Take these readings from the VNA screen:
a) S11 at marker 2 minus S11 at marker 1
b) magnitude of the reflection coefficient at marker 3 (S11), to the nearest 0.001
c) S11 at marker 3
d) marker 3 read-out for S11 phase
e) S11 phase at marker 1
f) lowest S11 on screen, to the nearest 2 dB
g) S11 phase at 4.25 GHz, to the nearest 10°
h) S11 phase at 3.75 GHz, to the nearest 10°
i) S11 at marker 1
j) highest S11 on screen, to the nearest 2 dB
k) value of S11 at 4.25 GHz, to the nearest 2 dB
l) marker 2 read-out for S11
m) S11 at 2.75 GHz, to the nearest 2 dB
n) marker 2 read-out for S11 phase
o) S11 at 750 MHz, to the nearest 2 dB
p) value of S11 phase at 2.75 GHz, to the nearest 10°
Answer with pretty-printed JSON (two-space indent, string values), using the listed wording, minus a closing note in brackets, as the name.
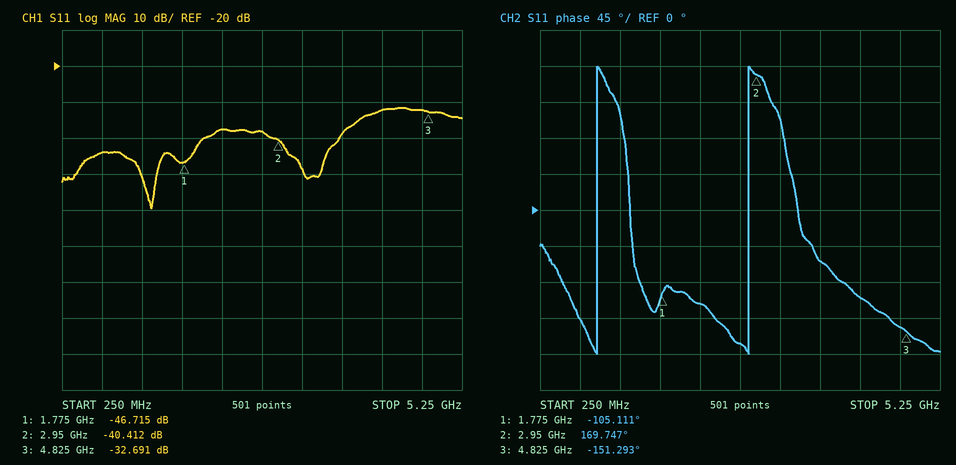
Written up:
{
  "S11 at marker 2 minus S11 at marker 1": "6.303 dB",
  "magnitude of the reflection coefficient at marker 3 (S11), to the nearest 0.001": "0.023",
  "S11 at marker 3": "-32.691 dB",
  "marker 3 read-out for S11 phase": "-151.293°",
  "S11 phase at marker 1": "-105.111°",
  "lowest S11 on screen, to the nearest 2 dB": "-60 dB",
  "S11 phase at 4.25 GHz, to the nearest 10°": "-110°",
  "S11 phase at 3.75 GHz, to the nearest 10°": "-60°",
  "S11 at marker 1": "-46.715 dB",
  "highest S11 on screen, to the nearest 2 dB": "-32 dB",
  "value of S11 at 4.25 GHz, to the nearest 2 dB": "-32 dB",
  "marker 2 read-out for S11": "-40.412 dB",
  "S11 at 2.75 GHz, to the nearest 2 dB": "-38 dB",
  "marker 2 read-out for S11 phase": "169.747°",
  "S11 at 750 MHz, to the nearest 2 dB": "-44 dB",
  "value of S11 phase at 2.75 GHz, to the nearest 10°": "-170°"
}
